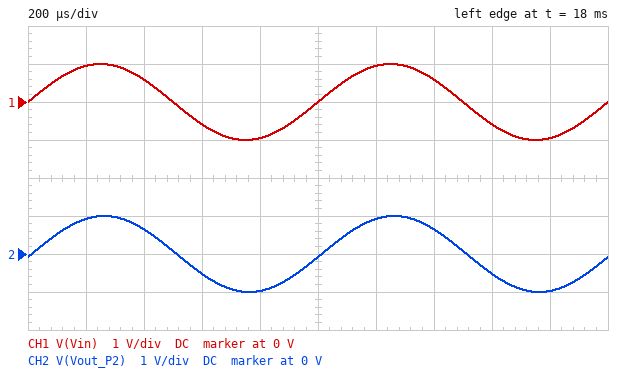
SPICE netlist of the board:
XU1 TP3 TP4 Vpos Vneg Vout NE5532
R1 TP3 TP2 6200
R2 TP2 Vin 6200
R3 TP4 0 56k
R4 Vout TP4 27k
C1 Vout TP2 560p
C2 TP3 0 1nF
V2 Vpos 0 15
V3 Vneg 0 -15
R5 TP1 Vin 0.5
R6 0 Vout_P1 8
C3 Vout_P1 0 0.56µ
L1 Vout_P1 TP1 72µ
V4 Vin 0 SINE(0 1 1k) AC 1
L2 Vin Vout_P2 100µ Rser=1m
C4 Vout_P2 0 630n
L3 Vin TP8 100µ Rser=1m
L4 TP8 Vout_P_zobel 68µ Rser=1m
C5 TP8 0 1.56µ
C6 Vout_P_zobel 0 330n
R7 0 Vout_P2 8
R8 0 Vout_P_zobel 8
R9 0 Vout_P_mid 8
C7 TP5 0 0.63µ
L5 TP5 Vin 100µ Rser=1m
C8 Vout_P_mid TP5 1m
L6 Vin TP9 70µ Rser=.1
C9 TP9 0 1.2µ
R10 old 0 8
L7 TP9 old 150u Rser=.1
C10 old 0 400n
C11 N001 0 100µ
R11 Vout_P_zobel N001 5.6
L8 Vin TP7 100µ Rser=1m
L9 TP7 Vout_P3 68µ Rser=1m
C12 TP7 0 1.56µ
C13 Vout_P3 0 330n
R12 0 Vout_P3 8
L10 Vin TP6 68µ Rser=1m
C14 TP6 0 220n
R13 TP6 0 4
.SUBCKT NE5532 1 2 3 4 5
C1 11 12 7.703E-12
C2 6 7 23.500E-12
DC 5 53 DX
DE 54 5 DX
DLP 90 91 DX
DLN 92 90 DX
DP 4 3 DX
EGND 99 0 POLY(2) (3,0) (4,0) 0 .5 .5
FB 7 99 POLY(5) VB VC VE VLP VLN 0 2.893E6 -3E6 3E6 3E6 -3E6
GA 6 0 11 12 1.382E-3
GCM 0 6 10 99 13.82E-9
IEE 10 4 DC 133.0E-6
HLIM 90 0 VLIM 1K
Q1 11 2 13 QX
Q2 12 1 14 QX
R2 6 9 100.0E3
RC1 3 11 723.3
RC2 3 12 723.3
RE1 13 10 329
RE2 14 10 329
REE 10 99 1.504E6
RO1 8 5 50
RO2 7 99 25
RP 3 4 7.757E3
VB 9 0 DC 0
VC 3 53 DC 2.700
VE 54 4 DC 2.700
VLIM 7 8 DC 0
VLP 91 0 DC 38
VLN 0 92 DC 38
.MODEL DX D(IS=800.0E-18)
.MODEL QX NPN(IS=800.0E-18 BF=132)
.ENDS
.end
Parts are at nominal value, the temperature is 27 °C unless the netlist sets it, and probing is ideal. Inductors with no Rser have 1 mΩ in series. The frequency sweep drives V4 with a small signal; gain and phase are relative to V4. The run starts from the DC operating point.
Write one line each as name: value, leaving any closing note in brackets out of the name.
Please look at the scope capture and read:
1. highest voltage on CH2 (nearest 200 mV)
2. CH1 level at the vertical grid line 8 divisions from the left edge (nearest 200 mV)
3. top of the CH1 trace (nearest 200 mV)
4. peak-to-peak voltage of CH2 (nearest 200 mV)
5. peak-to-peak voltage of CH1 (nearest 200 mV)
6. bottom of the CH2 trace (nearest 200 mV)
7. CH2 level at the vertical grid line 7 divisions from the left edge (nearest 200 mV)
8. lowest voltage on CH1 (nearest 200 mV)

highest voltage on CH2: 1.0 V
CH1 level at the vertical grid line 8 divisions from the left edge: -600 mV
top of the CH1 trace: 1.0 V
peak-to-peak voltage of CH2: 2.0 V
peak-to-peak voltage of CH1: 2.0 V
bottom of the CH2 trace: -1.0 V
CH2 level at the vertical grid line 7 divisions from the left edge: 600 mV
lowest voltage on CH1: -1.0 V
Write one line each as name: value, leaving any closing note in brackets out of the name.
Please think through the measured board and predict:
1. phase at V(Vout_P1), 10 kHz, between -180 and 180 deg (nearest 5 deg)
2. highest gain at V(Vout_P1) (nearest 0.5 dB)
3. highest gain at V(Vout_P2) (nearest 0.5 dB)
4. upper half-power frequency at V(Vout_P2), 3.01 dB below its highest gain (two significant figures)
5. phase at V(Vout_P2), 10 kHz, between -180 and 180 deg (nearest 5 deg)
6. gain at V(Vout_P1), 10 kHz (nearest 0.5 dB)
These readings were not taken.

phase at V(Vout_P1), 10 kHz, between -180 and 180 deg: -35 deg
highest gain at V(Vout_P1): -0.5 dB
highest gain at V(Vout_P2): 0 dB
upper half-power frequency at V(Vout_P2), 3.01 dB below its highest gain: 18 kHz
phase at V(Vout_P2), 10 kHz, between -180 and 180 deg: -45 deg
gain at V(Vout_P1), 10 kHz: -0.5 dB
